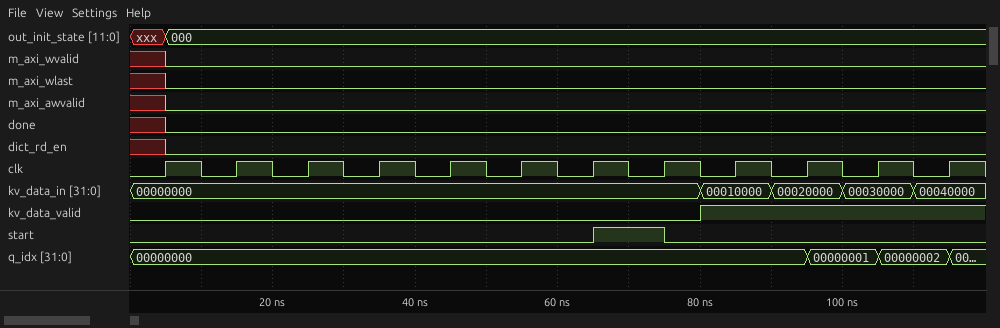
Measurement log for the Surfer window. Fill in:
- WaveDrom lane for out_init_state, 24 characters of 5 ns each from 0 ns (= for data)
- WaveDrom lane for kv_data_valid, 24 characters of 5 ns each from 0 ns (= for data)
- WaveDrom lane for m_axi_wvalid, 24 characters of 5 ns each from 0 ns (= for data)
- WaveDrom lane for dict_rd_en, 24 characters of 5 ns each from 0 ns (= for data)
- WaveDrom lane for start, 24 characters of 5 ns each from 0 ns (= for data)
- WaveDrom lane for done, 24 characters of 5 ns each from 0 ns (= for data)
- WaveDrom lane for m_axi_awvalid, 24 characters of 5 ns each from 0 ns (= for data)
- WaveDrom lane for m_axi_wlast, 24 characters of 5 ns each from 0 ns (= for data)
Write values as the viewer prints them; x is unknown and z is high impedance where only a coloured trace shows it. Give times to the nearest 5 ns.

{name: 'out_init_state', wave: 'x=......................', data: '000'}
{name: 'kv_data_valid', wave: '0...............1.......'}
{name: 'm_axi_wvalid', wave: 'x0......................'}
{name: 'dict_rd_en', wave: 'x0......................'}
{name: 'start', wave: '0............1.0........'}
{name: 'done', wave: 'x0......................'}
{name: 'm_axi_awvalid', wave: 'x0......................'}
{name: 'm_axi_wlast', wave: 'x0......................'}
